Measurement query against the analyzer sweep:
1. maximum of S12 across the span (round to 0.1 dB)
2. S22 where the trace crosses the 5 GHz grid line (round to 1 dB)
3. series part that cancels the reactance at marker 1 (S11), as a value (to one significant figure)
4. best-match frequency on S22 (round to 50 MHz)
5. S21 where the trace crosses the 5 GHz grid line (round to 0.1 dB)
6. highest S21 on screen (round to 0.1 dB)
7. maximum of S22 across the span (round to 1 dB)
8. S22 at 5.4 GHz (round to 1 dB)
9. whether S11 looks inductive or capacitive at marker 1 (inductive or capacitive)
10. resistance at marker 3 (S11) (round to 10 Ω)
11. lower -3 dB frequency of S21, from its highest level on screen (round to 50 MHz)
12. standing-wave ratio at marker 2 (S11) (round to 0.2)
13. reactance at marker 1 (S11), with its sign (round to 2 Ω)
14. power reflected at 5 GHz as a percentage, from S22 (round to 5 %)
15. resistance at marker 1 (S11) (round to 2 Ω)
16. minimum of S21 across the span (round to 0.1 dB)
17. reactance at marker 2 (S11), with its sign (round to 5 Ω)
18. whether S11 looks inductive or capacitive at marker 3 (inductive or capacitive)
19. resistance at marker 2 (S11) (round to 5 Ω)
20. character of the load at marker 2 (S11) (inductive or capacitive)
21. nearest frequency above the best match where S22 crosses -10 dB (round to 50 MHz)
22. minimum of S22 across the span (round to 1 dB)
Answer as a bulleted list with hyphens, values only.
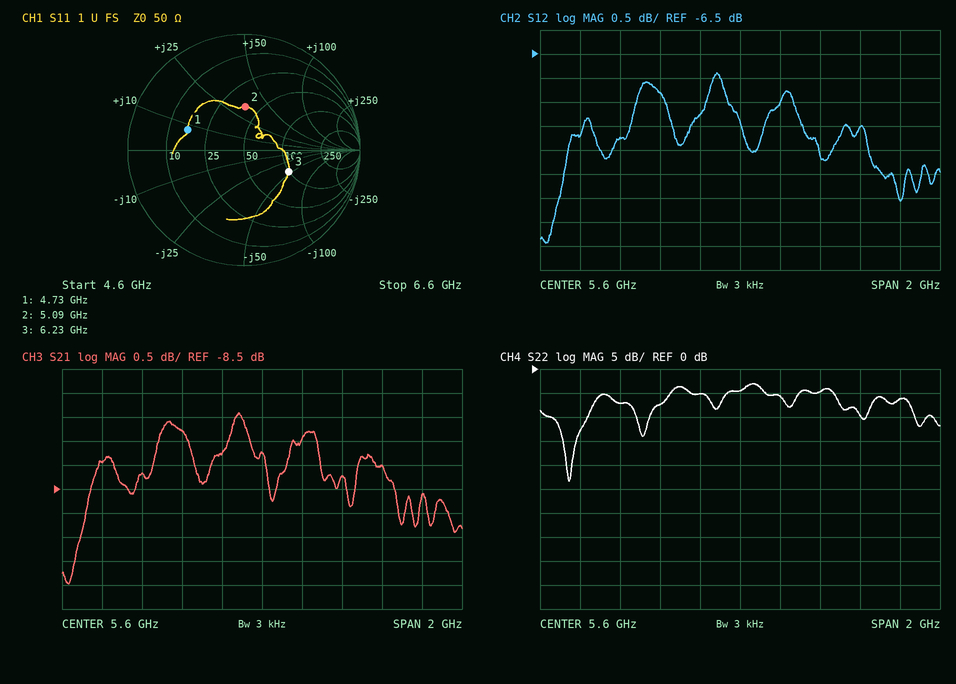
- -6.9 dB
- -7 dB
- 4 pF
- 4.75 GHz
- -8.2 dB
- -6.9 dB
- -3 dB
- -5 dB
- inductive
- 100 Ω
- 4.65 GHz
- 2.2
- +8 Ω
- 20 %
- 16 Ω
- -10.5 dB
- +35 Ω
- capacitive
- 40 Ω
- inductive
- 4.85 GHz
- -23 dB
